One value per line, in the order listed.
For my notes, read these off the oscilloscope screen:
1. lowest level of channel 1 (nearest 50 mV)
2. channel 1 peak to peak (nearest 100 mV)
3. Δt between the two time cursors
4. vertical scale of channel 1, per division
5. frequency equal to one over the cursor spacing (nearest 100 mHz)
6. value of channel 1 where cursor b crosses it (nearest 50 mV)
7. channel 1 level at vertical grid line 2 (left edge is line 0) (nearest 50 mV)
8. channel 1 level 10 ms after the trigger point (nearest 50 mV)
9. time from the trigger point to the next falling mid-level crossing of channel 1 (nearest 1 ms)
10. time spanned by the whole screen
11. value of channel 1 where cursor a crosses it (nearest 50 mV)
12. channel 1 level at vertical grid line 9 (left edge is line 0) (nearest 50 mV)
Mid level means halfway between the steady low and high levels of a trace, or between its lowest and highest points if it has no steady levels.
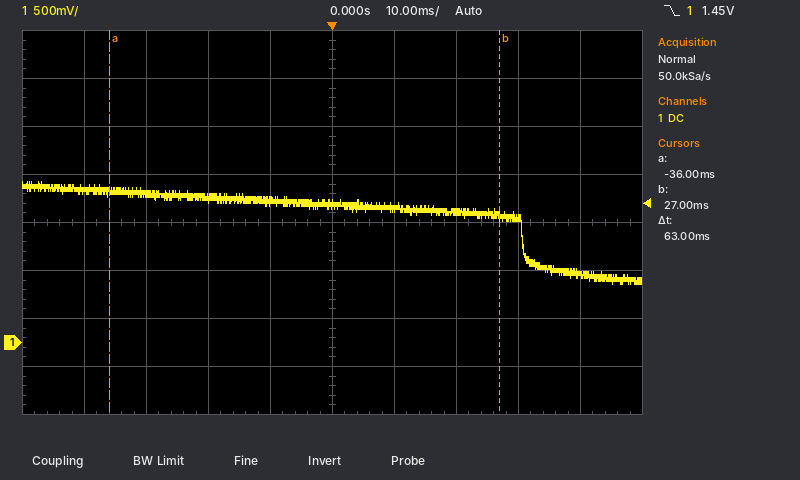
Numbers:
600 mV
1.10 V
63 ms
500 mV
15.9 Hz
1.30 V
1.55 V
1.40 V
31 ms
100 ms
1.55 V
700 mV
